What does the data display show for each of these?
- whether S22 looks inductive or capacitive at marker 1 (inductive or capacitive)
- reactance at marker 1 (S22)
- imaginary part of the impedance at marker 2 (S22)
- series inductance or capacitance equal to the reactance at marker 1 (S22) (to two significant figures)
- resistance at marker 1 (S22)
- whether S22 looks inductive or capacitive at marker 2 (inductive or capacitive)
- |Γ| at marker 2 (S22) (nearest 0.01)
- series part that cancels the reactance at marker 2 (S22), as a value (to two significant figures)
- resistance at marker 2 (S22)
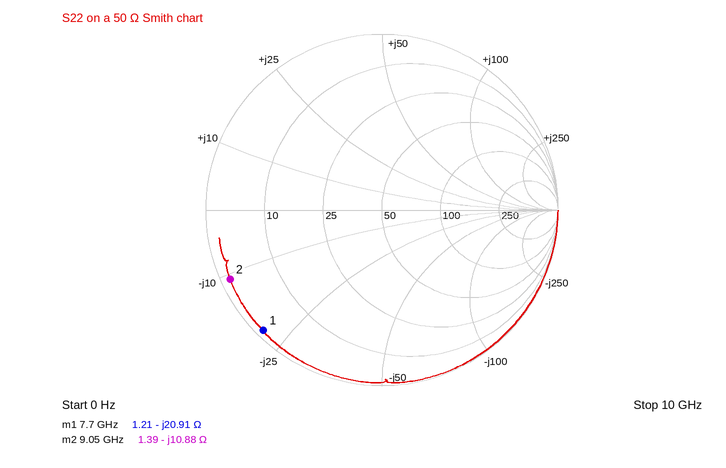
capacitive
-20.91 Ω
-10.88 Ω
990 fF
1.21 Ω
capacitive
0.95
190 pH
1.39 Ω
